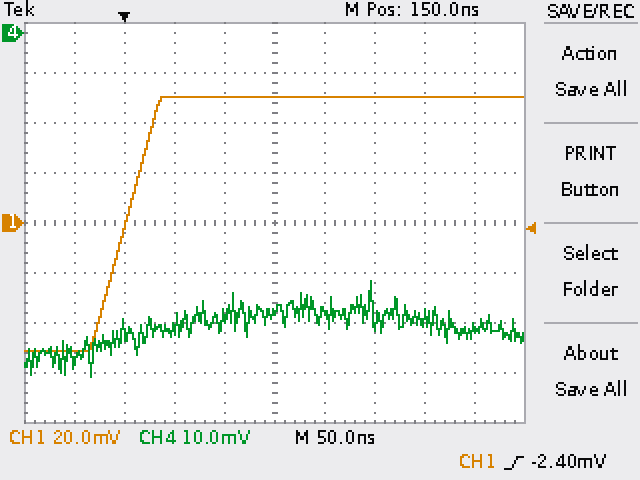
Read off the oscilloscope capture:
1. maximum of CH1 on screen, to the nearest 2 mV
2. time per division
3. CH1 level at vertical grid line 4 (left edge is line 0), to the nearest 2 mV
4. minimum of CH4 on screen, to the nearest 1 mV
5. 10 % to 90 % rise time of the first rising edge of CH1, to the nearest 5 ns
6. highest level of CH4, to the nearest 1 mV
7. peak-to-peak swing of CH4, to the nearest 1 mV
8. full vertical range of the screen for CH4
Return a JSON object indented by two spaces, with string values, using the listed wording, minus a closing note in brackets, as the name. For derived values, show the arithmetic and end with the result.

{
  "maximum of CH1 on screen, to the nearest 2 mV": "50 mV",
  "time per division": "50 ns",
  "CH1 level at vertical grid line 4 (left edge is line 0), to the nearest 2 mV": "50 mV",
  "minimum of CH4 on screen, to the nearest 1 mV": "-69 mV",
  "10 % to 90 % rise time of the first rising edge of CH1, to the nearest 5 ns": "55 ns",
  "highest level of CH4, to the nearest 1 mV": "-50 mV",
  "peak-to-peak swing of CH4, to the nearest 1 mV": "-50 mV − (-69 mV) = 19 mV",
  "full vertical range of the screen for CH4": "80 mV"
}
